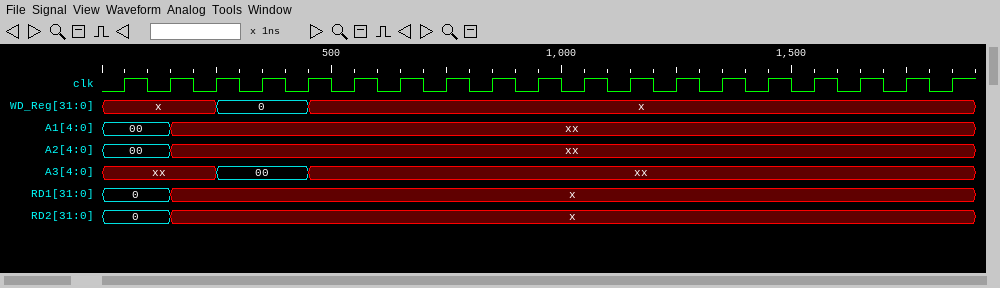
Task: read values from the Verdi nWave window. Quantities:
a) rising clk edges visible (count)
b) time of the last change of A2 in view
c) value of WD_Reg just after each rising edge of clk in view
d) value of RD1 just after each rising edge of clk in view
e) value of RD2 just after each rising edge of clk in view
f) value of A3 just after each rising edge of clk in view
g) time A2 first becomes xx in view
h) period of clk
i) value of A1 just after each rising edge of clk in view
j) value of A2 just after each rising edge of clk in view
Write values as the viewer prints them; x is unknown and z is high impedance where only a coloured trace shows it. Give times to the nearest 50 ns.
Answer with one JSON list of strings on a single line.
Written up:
["19", "150 ns", "x, x, 0, 0, x, x, x, x, x, x, x, x, x, x, x, x, x, x, x", "0, x, x, x, x, x, x, x, x, x, x, x, x, x, x, x, x, x, x", "0, x, x, x, x, x, x, x, x, x, x, x, x, x, x, x, x, x, x", "xx, xx, 00, 00, xx, xx, xx, xx, xx, xx, xx, xx, xx, xx, xx, xx, xx, xx, xx", "150 ns", "100 ns", "00, xx, xx, xx, xx, xx, xx, xx, xx, xx, xx, xx, xx, xx, xx, xx, xx, xx, xx", "00, xx, xx, xx, xx, xx, xx, xx, xx, xx, xx, xx, xx, xx, xx, xx, xx, xx, xx"]
